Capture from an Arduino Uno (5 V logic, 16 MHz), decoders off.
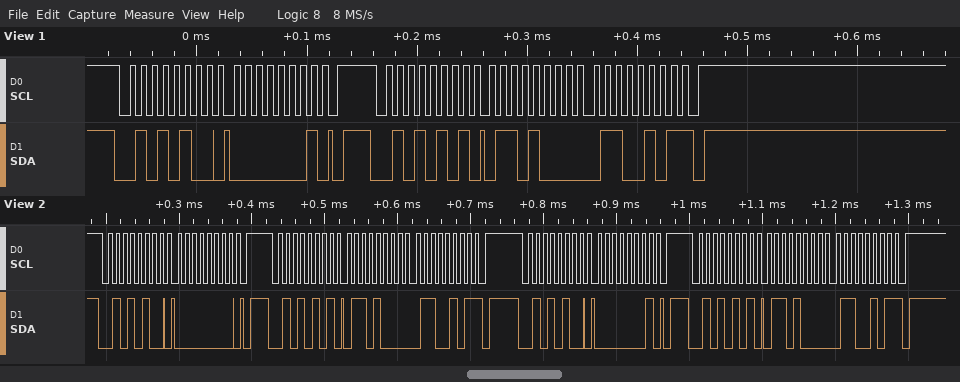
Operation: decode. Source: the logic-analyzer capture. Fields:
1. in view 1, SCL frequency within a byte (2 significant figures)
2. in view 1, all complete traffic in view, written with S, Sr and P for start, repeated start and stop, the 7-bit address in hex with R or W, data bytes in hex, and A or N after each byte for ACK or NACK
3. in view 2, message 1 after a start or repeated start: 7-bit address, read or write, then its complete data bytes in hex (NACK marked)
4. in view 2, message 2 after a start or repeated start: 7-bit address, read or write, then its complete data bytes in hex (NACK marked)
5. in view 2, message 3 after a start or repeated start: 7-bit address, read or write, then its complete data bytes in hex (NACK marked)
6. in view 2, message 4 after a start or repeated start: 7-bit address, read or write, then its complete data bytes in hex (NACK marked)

100 kHz
S 2AW A 01 A P S 2AR A 68 A 65 N P
0x2A write: 00
0x2A read: 68 65 NACK
0x2A write: 01
0x2A read: 68 65 NACK
